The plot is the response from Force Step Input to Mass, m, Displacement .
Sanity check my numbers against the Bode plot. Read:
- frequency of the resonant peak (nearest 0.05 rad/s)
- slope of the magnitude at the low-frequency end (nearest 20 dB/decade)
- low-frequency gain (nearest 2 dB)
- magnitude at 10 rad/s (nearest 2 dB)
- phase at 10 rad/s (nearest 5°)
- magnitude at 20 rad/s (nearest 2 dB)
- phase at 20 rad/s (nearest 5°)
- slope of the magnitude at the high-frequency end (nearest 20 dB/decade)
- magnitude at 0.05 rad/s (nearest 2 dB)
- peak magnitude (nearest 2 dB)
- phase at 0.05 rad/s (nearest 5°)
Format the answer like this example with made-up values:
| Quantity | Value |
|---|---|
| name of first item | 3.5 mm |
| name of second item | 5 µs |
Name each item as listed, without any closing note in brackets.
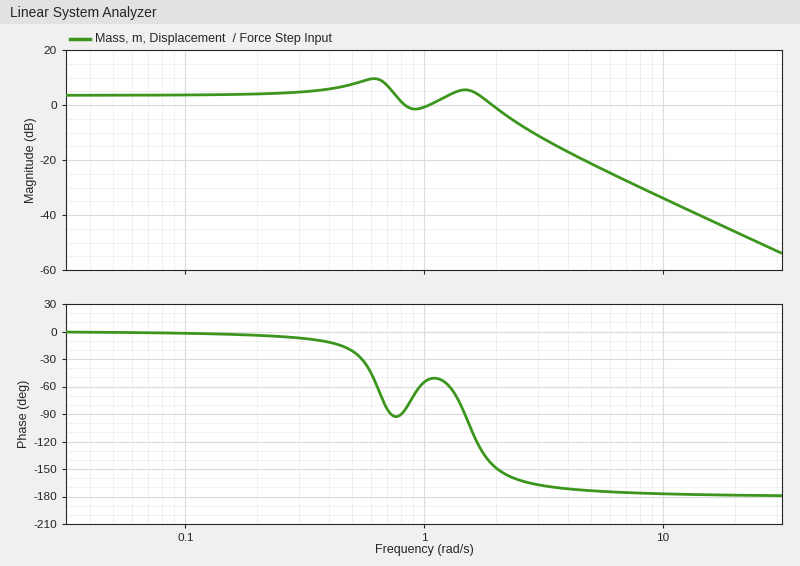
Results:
| Quantity | Value |
|---|---|
| frequency of the resonant peak | 0.60 rad/s |
| slope of the magnitude at the low-frequency end | 0 dB/decade |
| low-frequency gain | 4 dB |
| magnitude at 10 rad/s | -34 dB |
| phase at 10 rad/s | -175° |
| magnitude at 20 rad/s | -46 dB |
| phase at 20 rad/s | -180° |
| slope of the magnitude at the high-frequency end | -40 dB/decade |
| magnitude at 0.05 rad/s | 4 dB |
| peak magnitude | 10 dB |
| phase at 0.05 rad/s | 0° |
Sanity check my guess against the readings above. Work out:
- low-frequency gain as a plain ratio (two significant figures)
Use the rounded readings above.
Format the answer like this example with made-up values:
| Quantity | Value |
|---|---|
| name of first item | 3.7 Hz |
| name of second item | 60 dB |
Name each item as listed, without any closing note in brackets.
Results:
| Quantity | Value |
|---|---|
| low-frequency gain as a plain ratio | 1.6 |
